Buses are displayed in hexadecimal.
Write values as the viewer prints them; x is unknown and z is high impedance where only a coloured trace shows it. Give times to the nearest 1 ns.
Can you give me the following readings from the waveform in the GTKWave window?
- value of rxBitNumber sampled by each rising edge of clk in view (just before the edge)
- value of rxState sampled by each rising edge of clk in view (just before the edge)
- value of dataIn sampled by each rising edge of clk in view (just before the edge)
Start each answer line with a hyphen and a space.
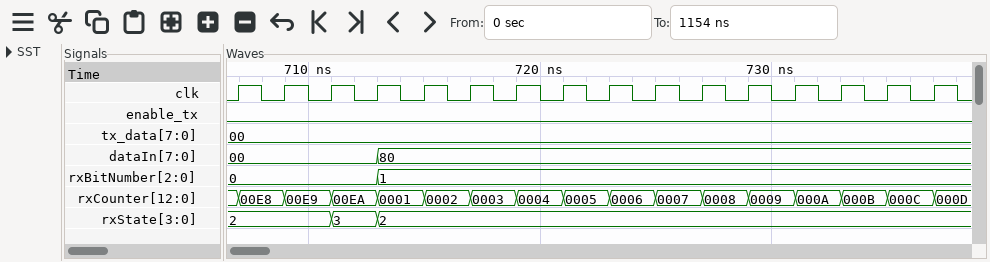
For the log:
- 0, 0, 0, 0, 1, 1, 1, 1, 1, 1, 1, 1, 1, 1, 1, 1
- 2, 2, 2, 3, 2, 2, 2, 2, 2, 2, 2, 2, 2, 2, 2, 2
- 00, 00, 00, 00, 80, 80, 80, 80, 80, 80, 80, 80, 80, 80, 80, 80
